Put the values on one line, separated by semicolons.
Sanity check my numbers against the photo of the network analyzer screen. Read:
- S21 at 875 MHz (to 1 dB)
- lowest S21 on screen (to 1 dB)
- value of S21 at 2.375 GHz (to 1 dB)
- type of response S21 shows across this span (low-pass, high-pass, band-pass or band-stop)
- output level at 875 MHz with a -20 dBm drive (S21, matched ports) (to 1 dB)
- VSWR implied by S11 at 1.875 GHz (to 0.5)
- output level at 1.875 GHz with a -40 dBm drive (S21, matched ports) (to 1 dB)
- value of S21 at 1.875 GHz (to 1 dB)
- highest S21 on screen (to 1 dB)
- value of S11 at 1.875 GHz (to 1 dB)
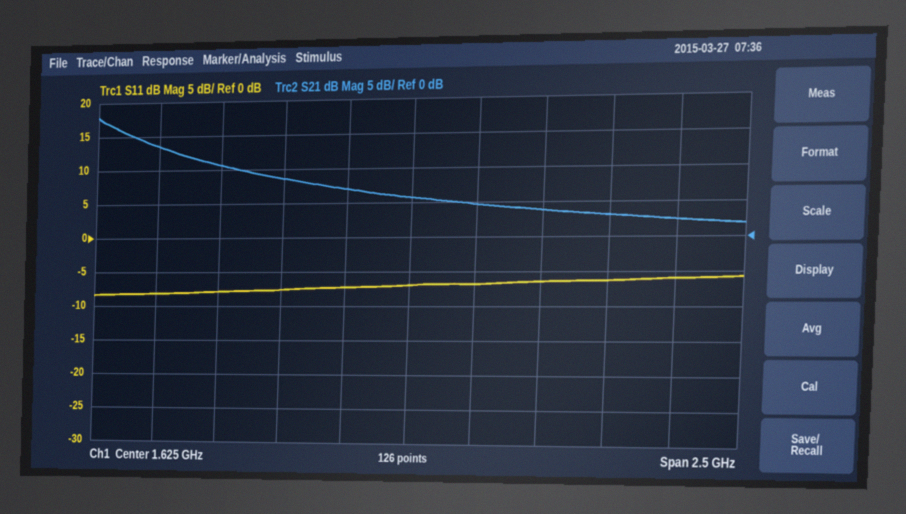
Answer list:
11 dB; 2 dB; 3 dB; low-pass; -9 dBm; 2.5; -35 dBm; 5 dB; 18 dB; -7 dB
